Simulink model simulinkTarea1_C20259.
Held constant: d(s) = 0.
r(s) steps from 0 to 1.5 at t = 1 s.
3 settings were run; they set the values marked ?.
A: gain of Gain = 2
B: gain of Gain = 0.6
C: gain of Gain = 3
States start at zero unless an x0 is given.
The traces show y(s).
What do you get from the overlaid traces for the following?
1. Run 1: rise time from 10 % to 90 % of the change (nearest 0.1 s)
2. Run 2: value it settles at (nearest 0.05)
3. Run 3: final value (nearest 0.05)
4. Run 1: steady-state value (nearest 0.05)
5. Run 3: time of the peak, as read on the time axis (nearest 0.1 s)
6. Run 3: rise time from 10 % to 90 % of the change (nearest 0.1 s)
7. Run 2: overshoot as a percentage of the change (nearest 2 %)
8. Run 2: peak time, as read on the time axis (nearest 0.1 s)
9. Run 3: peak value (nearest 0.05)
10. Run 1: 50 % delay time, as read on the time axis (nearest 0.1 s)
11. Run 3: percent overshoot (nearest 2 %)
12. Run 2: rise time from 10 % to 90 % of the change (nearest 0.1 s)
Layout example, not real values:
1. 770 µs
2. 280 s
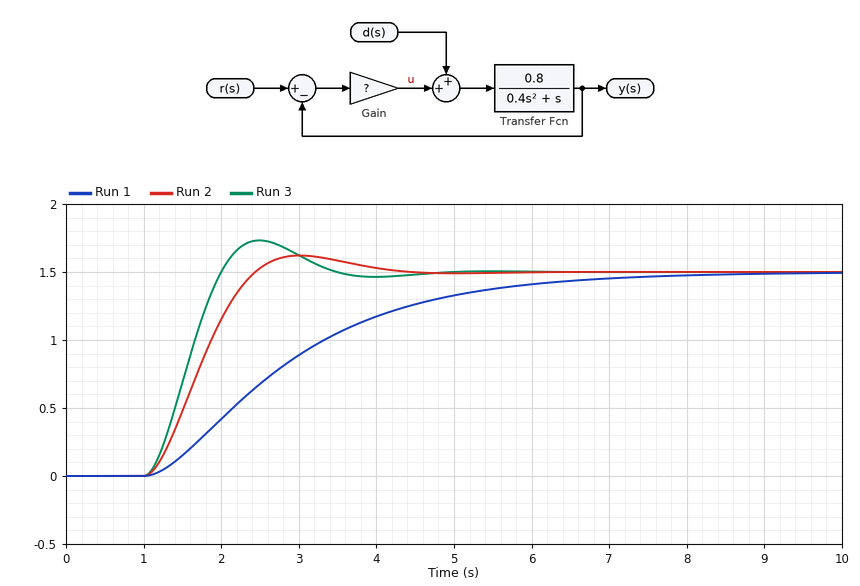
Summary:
1. 3.7 s
2. 1.50
3. 1.50
4. 1.50
5. 2.5 s
6. 0.7 s
7. 8 %
8. 3.0 s
9. 1.75
10. 2.7 s
11. 16 %
12. 1.0 s
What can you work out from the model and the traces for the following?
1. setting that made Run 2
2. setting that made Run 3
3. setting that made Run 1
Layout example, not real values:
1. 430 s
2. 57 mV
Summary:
1. A
2. C
3. B
